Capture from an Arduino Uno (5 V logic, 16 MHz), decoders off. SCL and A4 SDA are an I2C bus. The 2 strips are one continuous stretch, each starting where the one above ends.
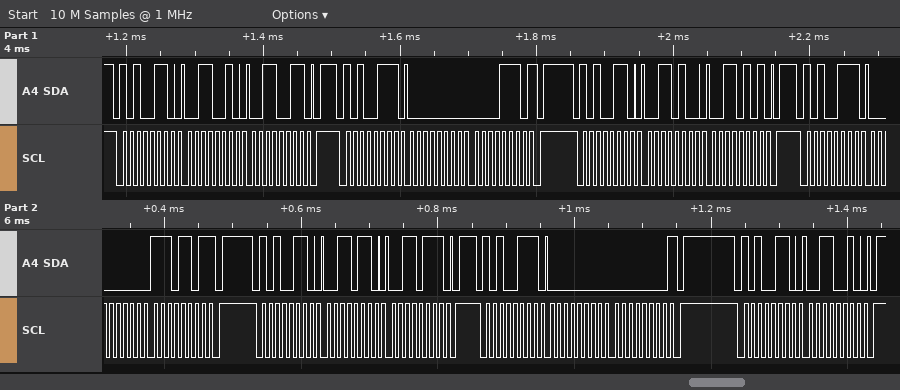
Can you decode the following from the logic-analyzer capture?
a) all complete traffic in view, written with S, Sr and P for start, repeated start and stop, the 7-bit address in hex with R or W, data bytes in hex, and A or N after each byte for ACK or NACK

S 53W A 32 A 33 A P S 53R A 00 A 0E N P S 53W A 34 A 35 A P S 53R A 00 A ED N P S 53W A 36 A 37 A P S 53R A 00 A 00 N P S 53W A 32 A P
